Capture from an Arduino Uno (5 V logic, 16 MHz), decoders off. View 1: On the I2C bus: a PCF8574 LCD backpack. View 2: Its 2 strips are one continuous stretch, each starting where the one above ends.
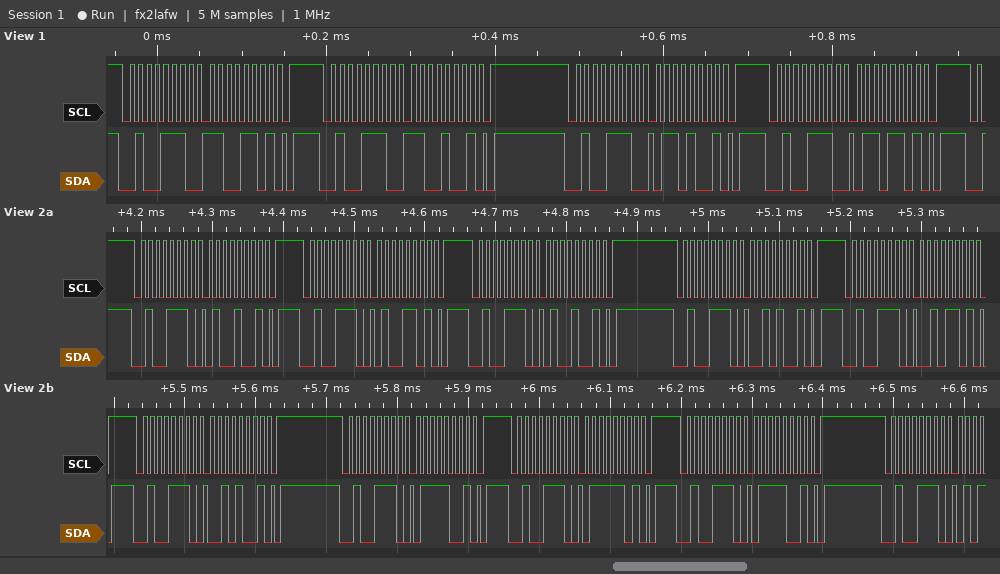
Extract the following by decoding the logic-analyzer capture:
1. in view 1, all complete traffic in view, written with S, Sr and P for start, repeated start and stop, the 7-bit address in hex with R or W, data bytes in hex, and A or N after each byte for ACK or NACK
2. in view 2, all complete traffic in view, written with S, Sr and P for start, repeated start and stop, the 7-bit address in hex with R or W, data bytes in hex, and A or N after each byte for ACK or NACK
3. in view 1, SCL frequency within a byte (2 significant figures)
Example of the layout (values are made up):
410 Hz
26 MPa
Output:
S 27W A CD A P S 27W A C9 A P S 27W A 69 A P S 27W A 6D A P
S 27W A 49 A P S 27W A 4D A P S 27W A 49 A P S 27W A 29 A P S 27W A 2D A P S 27W A 29 A P S 27W A 79 A P S 27W A 7D A P S 27W A 79 A P S 27W A
100 kHz
